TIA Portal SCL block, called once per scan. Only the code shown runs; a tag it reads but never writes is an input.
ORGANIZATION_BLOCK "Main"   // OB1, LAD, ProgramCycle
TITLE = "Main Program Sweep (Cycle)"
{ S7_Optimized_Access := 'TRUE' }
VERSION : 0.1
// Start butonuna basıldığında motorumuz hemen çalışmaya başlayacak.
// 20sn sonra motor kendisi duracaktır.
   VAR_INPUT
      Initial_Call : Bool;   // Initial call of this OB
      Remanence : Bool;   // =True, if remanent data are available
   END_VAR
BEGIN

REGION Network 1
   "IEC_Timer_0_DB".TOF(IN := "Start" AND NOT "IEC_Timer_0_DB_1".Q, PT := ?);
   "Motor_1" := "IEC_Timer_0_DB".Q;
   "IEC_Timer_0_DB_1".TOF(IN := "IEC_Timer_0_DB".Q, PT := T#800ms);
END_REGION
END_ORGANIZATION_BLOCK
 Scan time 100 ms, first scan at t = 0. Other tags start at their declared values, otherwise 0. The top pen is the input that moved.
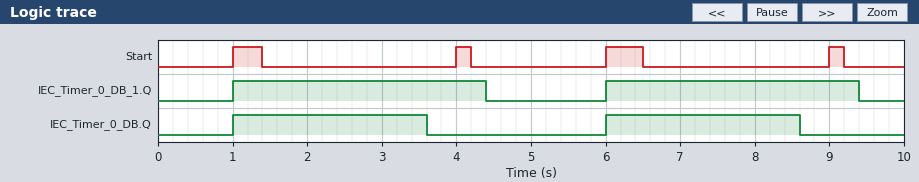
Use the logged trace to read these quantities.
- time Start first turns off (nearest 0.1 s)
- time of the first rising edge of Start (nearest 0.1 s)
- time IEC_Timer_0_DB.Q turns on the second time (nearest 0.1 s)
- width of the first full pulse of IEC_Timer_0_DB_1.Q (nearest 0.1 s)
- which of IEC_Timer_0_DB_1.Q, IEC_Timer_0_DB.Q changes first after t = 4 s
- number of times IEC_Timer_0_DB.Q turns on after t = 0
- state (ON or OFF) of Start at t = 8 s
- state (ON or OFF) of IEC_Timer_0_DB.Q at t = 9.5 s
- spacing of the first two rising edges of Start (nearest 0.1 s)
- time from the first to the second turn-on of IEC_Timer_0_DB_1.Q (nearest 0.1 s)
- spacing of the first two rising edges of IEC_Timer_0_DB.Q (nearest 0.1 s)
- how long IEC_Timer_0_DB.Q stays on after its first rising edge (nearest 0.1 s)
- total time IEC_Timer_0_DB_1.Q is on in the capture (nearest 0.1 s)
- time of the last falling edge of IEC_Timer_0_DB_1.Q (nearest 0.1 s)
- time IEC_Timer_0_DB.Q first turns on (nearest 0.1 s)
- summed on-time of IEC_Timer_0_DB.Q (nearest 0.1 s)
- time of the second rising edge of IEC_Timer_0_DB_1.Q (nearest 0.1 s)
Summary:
1.4 s
1.0 s
6.0 s
3.4 s
IEC_Timer_0_DB_1.Q
2
OFF
OFF
3.0 s
5.0 s
5.0 s
2.6 s
6.8 s
9.4 s
1.0 s
5.2 s
6.0 s
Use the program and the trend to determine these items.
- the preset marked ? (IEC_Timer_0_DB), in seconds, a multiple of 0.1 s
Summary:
2.5 s
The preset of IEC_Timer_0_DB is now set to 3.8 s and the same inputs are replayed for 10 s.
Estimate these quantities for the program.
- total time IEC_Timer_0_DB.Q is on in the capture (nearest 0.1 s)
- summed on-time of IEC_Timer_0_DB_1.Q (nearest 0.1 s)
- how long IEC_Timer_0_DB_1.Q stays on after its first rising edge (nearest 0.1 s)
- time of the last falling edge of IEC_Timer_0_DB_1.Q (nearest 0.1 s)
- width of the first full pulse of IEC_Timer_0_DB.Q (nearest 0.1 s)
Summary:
7.8 s
8.7 s
4.7 s
5.7 s
3.9 s
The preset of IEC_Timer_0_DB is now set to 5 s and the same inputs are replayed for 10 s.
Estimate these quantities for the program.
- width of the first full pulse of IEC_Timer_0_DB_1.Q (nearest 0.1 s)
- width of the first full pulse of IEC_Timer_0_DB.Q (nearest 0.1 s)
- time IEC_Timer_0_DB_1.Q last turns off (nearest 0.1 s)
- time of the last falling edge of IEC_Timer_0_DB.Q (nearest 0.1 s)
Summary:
5.9 s
5.1 s
6.9 s
6.1 s
